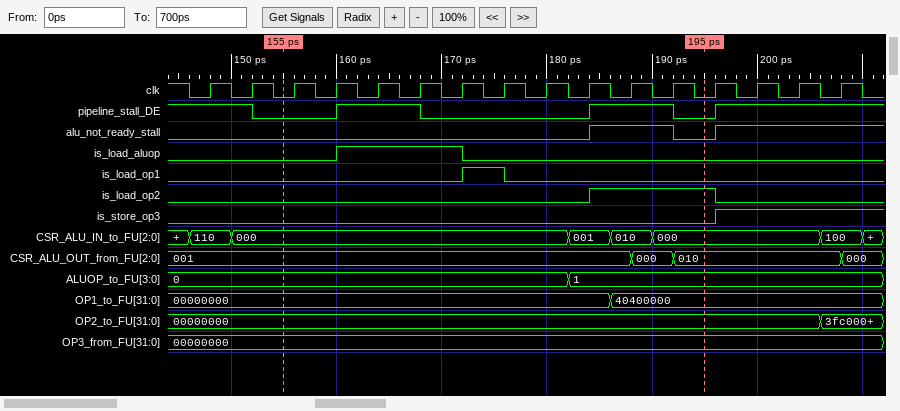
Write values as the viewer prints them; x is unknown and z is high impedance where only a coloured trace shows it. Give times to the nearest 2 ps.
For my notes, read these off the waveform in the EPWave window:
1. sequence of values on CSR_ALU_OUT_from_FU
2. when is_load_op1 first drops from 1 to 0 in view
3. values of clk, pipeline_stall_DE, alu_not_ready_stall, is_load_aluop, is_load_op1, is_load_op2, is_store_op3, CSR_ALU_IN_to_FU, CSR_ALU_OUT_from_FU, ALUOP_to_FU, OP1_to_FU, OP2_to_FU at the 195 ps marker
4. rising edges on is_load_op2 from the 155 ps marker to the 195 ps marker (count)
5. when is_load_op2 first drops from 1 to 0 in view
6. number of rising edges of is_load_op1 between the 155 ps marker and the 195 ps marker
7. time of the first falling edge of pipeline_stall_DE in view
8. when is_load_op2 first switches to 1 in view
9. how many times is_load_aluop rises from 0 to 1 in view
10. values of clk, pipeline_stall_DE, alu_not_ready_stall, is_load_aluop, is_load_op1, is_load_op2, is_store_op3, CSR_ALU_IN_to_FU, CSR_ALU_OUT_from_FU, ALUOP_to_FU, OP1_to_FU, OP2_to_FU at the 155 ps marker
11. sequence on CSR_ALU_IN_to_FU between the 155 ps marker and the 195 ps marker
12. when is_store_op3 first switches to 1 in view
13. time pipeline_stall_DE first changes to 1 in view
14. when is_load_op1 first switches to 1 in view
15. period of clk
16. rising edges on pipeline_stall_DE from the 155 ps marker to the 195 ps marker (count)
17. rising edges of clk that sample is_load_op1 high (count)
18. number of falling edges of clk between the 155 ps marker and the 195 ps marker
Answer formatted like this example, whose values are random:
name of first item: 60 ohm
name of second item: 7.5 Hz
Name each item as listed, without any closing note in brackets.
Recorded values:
sequence of values on CSR_ALU_OUT_from_FU: 001, 000, 010, 000
when is_load_op1 first drops from 1 to 0 in view: 176 ps
values of clk, pipeline_stall_DE, alu_not_ready_stall, is_load_aluop, is_load_op1, is_load_op2, is_store_op3, CSR_ALU_IN_to_FU, CSR_ALU_OUT_from_FU, ALUOP_to_FU, OP1_to_FU, OP2_to_FU at the 195 ps marker: clk=0, pipeline_stall_DE=0, alu_not_ready_stall=0, is_load_aluop=0, is_load_op1=0, is_load_op2=1, is_store_op3=0, CSR_ALU_IN_to_FU=000, CSR_ALU_OUT_from_FU=010, ALUOP_to_FU=1, OP1_to_FU=40400000, OP2_to_FU=00000000
rising edges on is_load_op2 from the 155 ps marker to the 195 ps marker: 1
when is_load_op2 first drops from 1 to 0 in view: 196 ps
number of rising edges of is_load_op1 between the 155 ps marker and the 195 ps marker: 1
time of the first falling edge of pipeline_stall_DE in view: 152 ps
when is_load_op2 first switches to 1 in view: 184 ps
how many times is_load_aluop rises from 0 to 1 in view: 1
values of clk, pipeline_stall_DE, alu_not_ready_stall, is_load_aluop, is_load_op1, is_load_op2, is_store_op3, CSR_ALU_IN_to_FU, CSR_ALU_OUT_from_FU, ALUOP_to_FU, OP1_to_FU, OP2_to_FU at the 155 ps marker: clk=0, pipeline_stall_DE=0, alu_not_ready_stall=0, is_load_aluop=0, is_load_op1=0, is_load_op2=0, is_store_op3=0, CSR_ALU_IN_to_FU=000, CSR_ALU_OUT_from_FU=001, ALUOP_to_FU=0, OP1_to_FU=00000000, OP2_to_FU=00000000
sequence on CSR_ALU_IN_to_FU between the 155 ps marker and the 195 ps marker: 000, 001, 010, 000
when is_store_op3 first switches to 1 in view: 196 ps
time pipeline_stall_DE first changes to 1 in view: 160 ps
when is_load_op1 first switches to 1 in view: 172 ps
period of clk: 4 ps
rising edges on pipeline_stall_DE from the 155 ps marker to the 195 ps marker: 2
rising edges of clk that sample is_load_op1 high: 1
number of falling edges of clk between the 155 ps marker and the 195 ps marker: 10
